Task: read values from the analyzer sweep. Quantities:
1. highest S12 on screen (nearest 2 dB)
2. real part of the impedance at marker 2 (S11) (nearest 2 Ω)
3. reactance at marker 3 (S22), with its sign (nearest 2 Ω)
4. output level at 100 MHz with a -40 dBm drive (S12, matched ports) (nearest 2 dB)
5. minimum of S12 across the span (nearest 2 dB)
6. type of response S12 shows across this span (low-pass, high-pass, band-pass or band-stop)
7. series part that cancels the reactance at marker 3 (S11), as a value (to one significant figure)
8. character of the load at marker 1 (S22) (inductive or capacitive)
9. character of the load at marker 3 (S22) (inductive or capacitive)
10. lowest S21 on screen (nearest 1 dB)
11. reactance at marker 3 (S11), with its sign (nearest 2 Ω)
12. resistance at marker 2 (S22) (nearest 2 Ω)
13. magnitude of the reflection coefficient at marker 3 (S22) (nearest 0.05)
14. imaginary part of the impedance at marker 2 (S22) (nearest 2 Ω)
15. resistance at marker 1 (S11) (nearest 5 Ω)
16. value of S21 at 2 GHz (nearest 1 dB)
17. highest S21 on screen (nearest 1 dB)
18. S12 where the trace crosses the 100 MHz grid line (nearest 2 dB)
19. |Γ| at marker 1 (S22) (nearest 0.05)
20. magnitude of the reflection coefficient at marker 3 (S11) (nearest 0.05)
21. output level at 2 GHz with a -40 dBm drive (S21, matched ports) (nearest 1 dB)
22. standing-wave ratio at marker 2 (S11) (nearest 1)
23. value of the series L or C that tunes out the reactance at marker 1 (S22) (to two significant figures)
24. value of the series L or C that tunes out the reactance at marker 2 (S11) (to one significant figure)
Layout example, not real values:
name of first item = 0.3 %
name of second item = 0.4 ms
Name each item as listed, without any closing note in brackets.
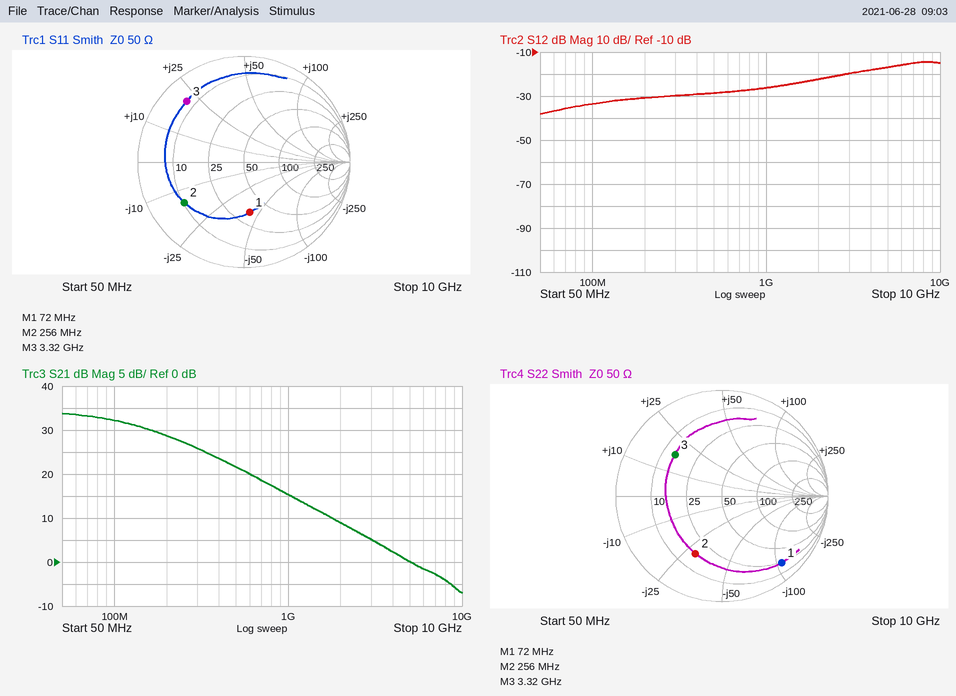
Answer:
highest S12 on screen = -14 dB
real part of the impedance at marker 2 (S11) = 10 Ω
reactance at marker 3 (S22), with its sign = +18 Ω
output level at 100 MHz with a -40 dBm drive (S12, matched ports) = -74 dBm
minimum of S12 across the span = -38 dB
type of response S12 shows across this span = high-pass
series part that cancels the reactance at marker 3 (S11), as a value = 2 pF
character of the load at marker 1 (S22) = capacitive
character of the load at marker 3 (S22) = inductive
lowest S21 on screen = -7 dB
reactance at marker 3 (S11), with its sign = +22 Ω
resistance at marker 2 (S22) = 18 Ω
magnitude of the reflection coefficient at marker 3 (S22) = 0.60
imaginary part of the impedance at marker 2 (S22) = -30 Ω
resistance at marker 1 (S11) = 35 Ω
value of S21 at 2 GHz = 9 dB
highest S21 on screen = 34 dB
S12 where the trace crosses the 100 MHz grid line = -34 dB
|Γ| at marker 1 (S22) = 0.85
magnitude of the reflection coefficient at marker 3 (S11) = 0.80
output level at 2 GHz with a -40 dBm drive (S21, matched ports) = -31 dBm
standing-wave ratio at marker 2 (S11) = 5
value of the series L or C that tunes out the reactance at marker 1 (S22) = 240 nH
value of the series L or C that tunes out the reactance at marker 2 (S11) = 9 nH
